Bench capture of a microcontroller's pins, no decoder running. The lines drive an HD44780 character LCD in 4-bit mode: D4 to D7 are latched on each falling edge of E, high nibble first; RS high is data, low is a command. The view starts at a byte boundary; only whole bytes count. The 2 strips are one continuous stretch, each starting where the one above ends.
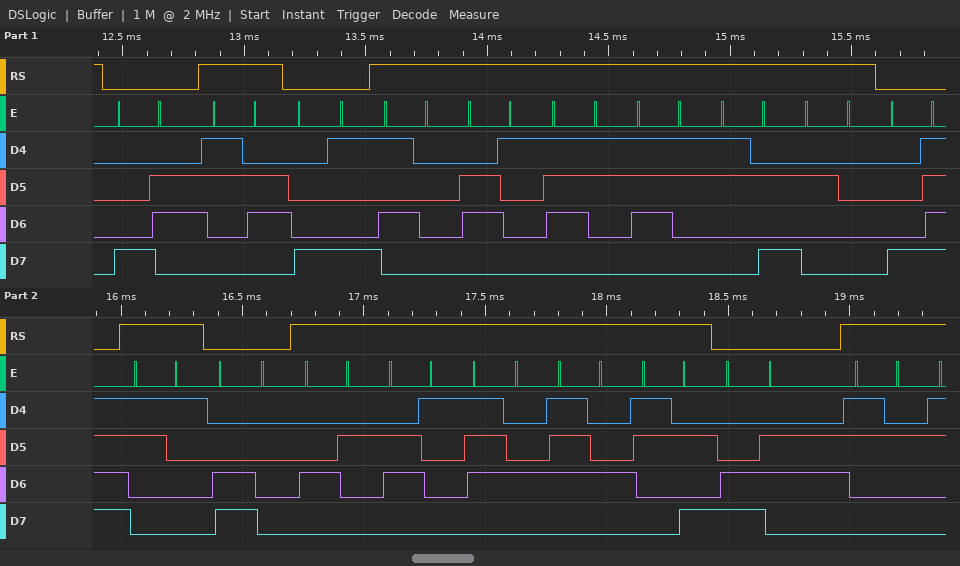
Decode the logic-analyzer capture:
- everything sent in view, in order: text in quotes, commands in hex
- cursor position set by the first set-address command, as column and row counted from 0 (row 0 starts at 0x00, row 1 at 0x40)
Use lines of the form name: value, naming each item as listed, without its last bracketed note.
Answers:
everything sent in view, in order: text in quotes, commands in hex: 0x86 "6" 0x89 "Pass: " 0x8F "1" 0xC0 "Batt:" 0xC6 "2"
cursor position set by the first set-address command, as column and row counted from 0: column 6, row 0
